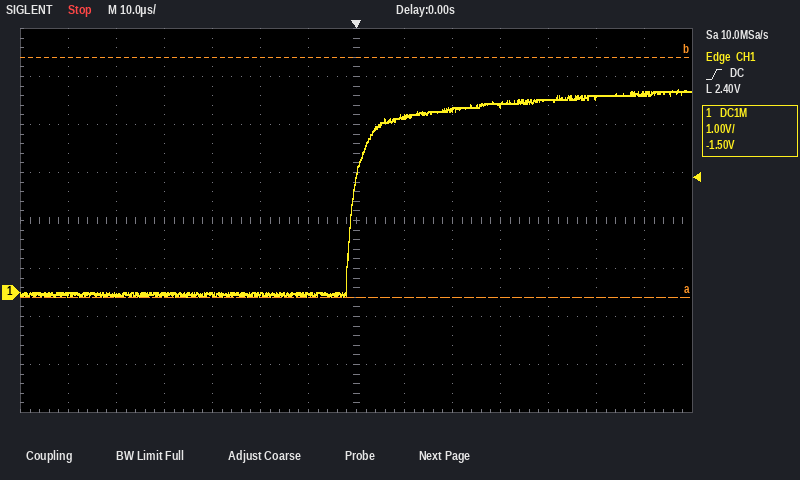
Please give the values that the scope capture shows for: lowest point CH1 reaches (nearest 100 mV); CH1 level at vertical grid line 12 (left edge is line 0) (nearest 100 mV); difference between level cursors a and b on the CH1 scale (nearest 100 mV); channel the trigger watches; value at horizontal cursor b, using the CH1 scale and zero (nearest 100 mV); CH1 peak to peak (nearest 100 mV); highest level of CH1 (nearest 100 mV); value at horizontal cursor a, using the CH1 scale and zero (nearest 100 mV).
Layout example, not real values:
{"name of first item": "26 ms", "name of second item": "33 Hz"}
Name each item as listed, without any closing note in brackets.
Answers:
{"lowest point CH1 reaches": "-100 mV", "CH1 level at vertical grid line 12 (left edge is line 0)": "4.1 V", "difference between level cursors a and b on the CH1 scale": "5.0 V", "channel the trigger watches": "CH1", "value at horizontal cursor b, using the CH1 scale and zero": "4.9 V", "CH1 peak to peak": "4.3 V", "highest level of CH1": "4.2 V", "value at horizontal cursor a, using the CH1 scale and zero": "-100 mV"}
